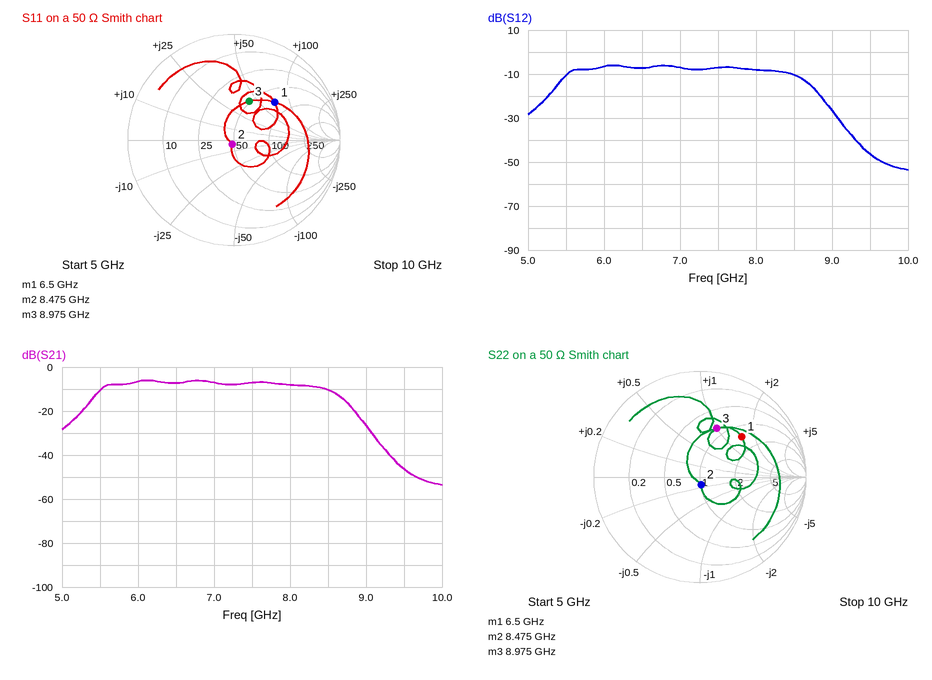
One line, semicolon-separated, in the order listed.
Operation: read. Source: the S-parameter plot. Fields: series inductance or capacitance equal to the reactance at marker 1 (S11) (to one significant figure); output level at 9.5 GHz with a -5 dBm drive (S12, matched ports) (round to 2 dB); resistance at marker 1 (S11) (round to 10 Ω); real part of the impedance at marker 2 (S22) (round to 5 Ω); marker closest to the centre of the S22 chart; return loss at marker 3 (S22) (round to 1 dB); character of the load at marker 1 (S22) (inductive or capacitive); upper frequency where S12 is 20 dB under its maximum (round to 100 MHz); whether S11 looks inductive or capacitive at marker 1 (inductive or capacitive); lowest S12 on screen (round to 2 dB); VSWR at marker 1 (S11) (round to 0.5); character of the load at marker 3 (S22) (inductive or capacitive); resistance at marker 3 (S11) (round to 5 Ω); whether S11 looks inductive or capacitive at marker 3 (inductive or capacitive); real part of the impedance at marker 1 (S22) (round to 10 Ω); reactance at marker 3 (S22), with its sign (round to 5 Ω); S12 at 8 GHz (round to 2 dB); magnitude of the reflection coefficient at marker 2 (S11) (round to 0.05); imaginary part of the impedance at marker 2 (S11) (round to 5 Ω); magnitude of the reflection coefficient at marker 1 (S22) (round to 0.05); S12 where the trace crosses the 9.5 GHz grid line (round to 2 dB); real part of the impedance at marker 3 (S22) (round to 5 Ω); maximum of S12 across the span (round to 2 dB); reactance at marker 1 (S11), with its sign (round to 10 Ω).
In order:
2 nH; -52 dBm; 70 Ω; 50 Ω; marker 2; 6 dB; inductive; 9.0 GHz; inductive; -54 dB; 3.0; inductive; 50 Ω; inductive; 70 Ω; +50 Ω; -8 dB; 0.05; -5 Ω; 0.55; -46 dB; 40 Ω; -6 dB; +70 Ω
